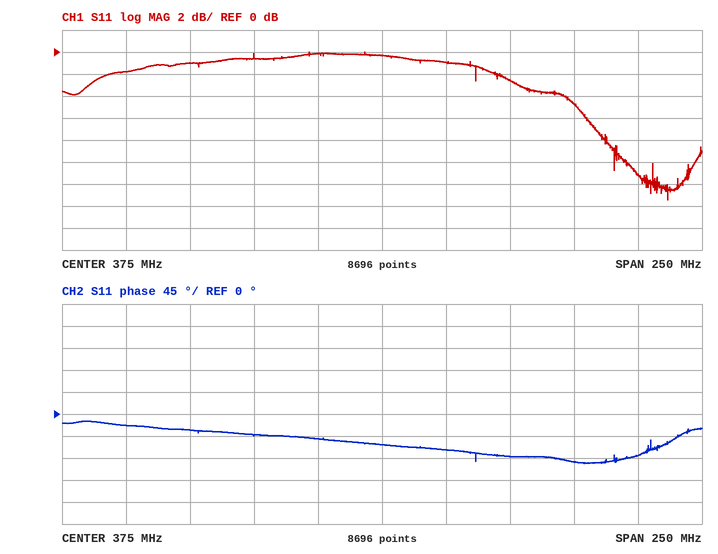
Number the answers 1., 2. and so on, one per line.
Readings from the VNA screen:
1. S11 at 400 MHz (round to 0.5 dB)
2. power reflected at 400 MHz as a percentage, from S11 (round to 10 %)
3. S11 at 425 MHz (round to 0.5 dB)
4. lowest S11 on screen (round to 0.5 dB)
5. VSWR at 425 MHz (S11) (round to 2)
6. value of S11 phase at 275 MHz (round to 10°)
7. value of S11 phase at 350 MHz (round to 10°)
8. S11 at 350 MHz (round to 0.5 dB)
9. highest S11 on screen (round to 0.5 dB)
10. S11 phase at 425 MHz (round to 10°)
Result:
1. -1.0 dB
2. 80 %
3. -2.5 dB
4. -13.5 dB
5. 6
6. -20°
7. -50°
8. 0.0 dB
9. 0.0 dB
10. -90°
